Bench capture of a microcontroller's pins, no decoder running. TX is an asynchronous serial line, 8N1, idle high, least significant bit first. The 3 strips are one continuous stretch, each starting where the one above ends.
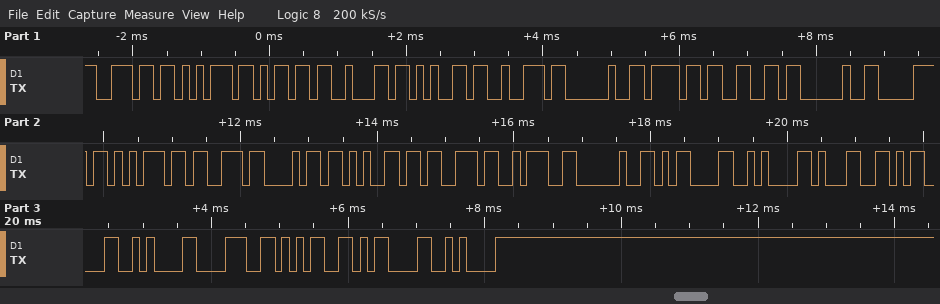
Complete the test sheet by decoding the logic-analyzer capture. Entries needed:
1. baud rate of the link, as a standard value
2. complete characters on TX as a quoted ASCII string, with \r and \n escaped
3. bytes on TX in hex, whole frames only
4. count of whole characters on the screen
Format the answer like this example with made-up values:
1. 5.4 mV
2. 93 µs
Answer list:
1. 9600 baud
2. "number of pushes: \r\n1\r\n85\r\n"
3. 6E 75 6D 62 65 72 20 6F 66 20 70 75 73 68 65 73 3A 20 0D 0A 31 0D 0A 38 35 0D 0A
4. 27
